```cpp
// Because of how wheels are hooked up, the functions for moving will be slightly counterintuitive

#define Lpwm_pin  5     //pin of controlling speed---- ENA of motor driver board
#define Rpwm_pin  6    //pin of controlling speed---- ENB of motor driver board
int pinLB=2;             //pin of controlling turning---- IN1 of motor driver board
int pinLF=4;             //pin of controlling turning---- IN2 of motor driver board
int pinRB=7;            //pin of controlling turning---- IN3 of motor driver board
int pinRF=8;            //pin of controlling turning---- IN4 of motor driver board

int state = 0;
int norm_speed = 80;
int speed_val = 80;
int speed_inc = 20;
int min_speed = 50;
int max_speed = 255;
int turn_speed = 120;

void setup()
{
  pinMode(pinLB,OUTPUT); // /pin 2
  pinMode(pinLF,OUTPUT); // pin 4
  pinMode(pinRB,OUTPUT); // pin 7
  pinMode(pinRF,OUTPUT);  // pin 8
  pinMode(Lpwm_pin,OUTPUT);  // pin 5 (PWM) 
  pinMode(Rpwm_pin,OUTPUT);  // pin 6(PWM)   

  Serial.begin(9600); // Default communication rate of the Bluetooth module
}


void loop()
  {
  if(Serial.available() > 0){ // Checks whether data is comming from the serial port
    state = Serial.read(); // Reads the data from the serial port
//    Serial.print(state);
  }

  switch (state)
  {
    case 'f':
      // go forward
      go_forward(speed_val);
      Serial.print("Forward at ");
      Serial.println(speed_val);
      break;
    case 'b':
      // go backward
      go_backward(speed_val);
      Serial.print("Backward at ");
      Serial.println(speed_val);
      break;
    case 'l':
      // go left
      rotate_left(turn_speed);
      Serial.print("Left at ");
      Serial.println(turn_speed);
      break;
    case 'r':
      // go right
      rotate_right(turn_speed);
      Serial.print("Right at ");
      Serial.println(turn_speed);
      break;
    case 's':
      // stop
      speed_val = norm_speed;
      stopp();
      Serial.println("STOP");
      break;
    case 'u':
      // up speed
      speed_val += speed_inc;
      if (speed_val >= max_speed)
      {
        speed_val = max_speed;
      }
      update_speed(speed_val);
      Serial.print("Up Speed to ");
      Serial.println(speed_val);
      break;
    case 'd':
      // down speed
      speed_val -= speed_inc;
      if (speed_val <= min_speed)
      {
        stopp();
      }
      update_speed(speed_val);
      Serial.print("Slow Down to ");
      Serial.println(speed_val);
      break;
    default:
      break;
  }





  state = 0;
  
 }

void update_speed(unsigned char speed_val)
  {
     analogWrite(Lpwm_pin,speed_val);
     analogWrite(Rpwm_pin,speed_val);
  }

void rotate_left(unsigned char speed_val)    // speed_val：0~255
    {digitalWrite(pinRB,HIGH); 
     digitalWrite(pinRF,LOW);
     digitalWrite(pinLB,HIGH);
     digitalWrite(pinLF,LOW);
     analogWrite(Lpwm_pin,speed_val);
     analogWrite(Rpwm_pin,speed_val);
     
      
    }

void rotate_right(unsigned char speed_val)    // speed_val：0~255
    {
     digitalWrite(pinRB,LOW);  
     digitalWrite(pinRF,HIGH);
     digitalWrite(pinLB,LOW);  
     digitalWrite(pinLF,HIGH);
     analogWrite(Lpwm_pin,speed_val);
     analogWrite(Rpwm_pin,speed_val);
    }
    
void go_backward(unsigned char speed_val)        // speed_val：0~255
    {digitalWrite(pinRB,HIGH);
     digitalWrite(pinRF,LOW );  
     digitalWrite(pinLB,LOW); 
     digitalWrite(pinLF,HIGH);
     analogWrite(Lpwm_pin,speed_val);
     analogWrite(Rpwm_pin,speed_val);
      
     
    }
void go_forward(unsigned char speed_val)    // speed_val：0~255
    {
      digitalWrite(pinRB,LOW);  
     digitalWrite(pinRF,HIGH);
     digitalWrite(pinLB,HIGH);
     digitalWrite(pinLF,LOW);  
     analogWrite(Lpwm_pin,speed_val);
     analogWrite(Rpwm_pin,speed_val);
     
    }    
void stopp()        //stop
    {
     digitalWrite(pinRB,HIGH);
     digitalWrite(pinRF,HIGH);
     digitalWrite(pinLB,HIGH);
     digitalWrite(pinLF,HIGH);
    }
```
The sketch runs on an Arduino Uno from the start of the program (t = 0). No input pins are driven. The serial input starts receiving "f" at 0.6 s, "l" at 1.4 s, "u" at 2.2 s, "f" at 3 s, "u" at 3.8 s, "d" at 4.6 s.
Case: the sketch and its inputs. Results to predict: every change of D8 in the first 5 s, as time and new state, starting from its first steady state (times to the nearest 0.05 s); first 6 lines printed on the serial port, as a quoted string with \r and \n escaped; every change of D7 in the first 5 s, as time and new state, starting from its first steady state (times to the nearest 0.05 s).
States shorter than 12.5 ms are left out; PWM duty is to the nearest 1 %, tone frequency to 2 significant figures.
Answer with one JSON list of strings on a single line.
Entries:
["0 s low; 0.6 s high; 1.4 s low; 3 s high", "\"Forward at 80\\r\\nLeft at 120\\r\\nUp Speed to 100\\r\\nForward at 100\\r\\nUp Speed to 120\\r\\nSlow Down to 100\\r\\n\"", "0 s low; 1.4 s high; 3 s low"]
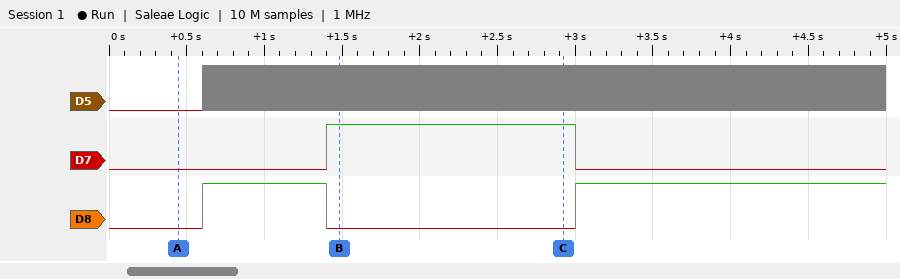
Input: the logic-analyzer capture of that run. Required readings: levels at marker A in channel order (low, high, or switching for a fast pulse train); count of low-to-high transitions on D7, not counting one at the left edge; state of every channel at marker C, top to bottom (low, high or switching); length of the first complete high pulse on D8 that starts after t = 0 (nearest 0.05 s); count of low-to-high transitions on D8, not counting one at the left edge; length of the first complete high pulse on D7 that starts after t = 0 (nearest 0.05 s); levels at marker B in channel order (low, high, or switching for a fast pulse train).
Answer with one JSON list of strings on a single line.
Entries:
["D5 low, D7 low, D8 low", "1", "D5 switching, D7 high, D8 low", "0.80 s", "2", "1.60 s", "D5 switching, D7 high, D8 low"]
